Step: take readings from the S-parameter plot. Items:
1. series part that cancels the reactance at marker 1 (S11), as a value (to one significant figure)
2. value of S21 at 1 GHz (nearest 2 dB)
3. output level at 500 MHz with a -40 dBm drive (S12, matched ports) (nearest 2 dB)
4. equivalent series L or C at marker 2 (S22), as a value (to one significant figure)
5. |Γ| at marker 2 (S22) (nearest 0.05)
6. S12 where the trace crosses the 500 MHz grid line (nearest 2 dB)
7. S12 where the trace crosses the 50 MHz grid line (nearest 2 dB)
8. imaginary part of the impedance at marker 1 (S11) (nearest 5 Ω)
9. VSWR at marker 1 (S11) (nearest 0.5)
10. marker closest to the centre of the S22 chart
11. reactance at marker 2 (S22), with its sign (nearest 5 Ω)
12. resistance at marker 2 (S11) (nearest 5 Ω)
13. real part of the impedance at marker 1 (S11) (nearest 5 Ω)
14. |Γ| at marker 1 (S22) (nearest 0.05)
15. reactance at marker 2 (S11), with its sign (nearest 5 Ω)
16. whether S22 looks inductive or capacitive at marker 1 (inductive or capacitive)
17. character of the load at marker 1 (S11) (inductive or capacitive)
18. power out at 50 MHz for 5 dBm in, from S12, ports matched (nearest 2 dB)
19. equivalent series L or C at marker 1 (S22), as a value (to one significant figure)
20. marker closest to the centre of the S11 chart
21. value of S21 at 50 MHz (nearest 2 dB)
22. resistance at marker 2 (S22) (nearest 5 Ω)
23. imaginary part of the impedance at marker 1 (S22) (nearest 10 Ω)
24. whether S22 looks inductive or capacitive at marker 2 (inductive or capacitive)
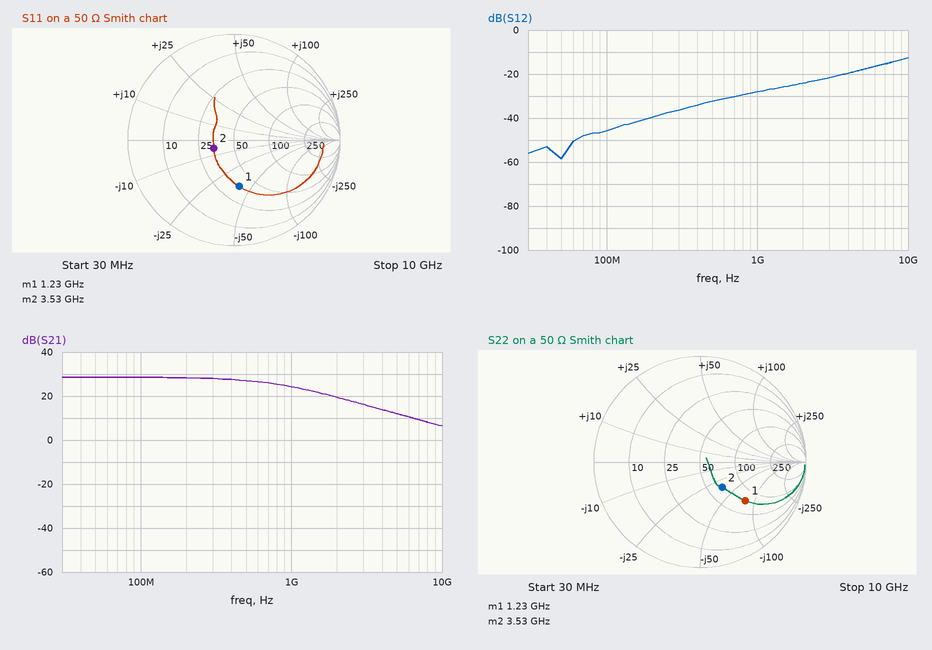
5 nH
24 dB
-72 dBm
1 pF
0.30
-32 dB
-58 dB
-40 Ω
2.5
marker 2
-35 Ω
35 Ω
35 Ω
0.55
-5 Ω
capacitive
capacitive
-54 dBm
2 pF
marker 2
28 dB
65 Ω
-80 Ω
capacitive
